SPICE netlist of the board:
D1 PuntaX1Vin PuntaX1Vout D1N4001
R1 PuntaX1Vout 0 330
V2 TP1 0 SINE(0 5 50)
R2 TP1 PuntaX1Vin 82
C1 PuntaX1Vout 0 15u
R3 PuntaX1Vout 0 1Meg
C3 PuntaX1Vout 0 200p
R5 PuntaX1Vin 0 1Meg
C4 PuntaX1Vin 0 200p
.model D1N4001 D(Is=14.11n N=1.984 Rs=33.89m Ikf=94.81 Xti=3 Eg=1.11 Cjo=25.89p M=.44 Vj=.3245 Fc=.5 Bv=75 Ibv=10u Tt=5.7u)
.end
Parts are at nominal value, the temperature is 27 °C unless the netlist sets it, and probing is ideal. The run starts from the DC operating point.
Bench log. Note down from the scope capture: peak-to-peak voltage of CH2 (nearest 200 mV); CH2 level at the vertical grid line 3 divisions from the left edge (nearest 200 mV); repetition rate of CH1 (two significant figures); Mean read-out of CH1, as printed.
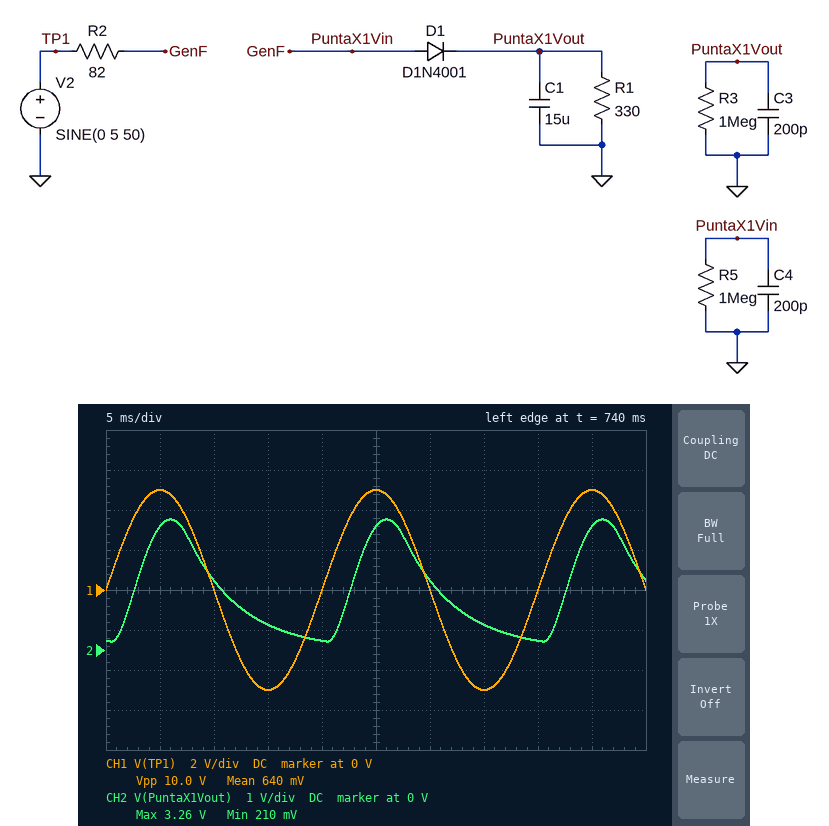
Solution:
3.0 V
600 mV
50 Hz
640 mV
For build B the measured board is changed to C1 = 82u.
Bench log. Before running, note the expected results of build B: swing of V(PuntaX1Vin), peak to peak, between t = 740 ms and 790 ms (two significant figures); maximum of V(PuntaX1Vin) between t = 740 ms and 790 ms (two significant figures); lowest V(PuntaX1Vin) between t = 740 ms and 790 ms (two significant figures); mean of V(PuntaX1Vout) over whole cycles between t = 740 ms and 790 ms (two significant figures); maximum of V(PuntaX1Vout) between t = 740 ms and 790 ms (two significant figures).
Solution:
8.1 V
3.1 V
-5.0 V
1.9 V
2.4 V
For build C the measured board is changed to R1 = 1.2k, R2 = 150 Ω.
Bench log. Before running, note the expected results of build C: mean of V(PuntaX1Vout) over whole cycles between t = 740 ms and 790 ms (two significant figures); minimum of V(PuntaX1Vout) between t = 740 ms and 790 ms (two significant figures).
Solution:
2.4 V
1.5 V
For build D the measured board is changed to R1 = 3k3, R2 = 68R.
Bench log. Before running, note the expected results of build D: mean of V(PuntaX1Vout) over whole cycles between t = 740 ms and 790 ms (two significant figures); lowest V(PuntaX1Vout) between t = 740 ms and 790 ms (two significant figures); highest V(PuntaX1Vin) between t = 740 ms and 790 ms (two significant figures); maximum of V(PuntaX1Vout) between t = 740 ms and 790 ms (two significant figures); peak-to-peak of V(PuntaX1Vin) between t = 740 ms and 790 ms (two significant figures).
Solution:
3.5 V
2.9 V
4.7 V
4.1 V
9.7 V
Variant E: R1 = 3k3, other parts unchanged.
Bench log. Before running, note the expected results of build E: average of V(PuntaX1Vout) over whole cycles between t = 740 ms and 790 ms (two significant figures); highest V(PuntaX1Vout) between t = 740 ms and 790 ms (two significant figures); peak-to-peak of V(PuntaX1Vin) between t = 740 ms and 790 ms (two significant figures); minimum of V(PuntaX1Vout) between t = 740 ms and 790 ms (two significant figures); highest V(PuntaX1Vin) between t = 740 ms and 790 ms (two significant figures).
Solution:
3.4 V
4.0 V
9.6 V
2.9 V
4.6 V
